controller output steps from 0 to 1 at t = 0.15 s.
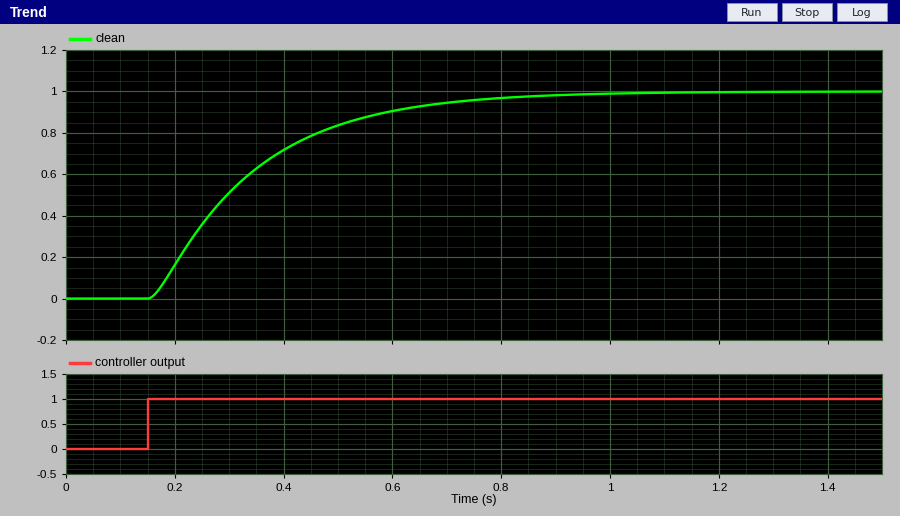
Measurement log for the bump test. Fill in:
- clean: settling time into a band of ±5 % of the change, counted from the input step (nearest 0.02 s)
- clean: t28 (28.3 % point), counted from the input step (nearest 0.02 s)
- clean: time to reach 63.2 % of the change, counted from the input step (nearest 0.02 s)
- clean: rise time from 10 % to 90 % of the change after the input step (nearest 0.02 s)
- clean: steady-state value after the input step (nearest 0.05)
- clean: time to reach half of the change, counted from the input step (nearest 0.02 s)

0.56 s
0.08 s
0.20 s
0.40 s
1.00
0.14 s
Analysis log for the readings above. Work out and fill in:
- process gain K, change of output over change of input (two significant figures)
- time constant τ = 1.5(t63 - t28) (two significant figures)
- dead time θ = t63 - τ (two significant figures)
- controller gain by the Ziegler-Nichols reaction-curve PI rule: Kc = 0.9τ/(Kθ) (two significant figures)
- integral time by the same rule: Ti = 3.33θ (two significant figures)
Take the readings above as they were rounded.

1.0
0.18 s
0.020 s
8.1
0.067 s
